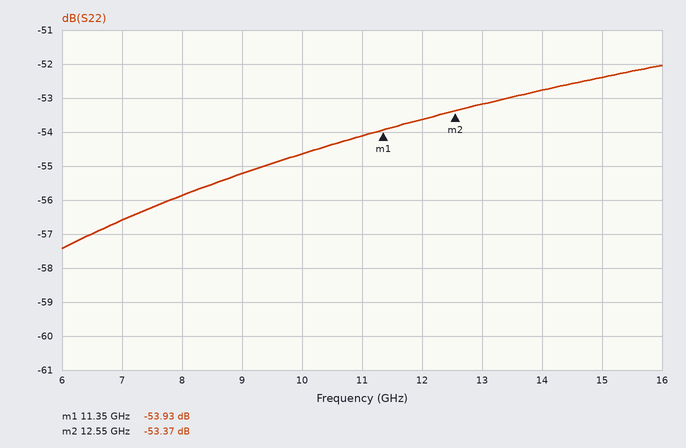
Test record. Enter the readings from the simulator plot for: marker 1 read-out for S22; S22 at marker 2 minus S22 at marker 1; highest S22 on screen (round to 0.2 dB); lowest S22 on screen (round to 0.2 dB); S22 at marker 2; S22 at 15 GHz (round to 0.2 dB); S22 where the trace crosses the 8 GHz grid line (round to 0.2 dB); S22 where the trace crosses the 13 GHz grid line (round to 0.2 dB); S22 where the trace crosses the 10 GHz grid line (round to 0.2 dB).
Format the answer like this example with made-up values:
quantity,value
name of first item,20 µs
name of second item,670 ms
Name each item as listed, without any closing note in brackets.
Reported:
quantity,value
marker 1 read-out for S22,-53.93 dB
S22 at marker 2 minus S22 at marker 1,0.56 dB
highest S22 on screen,-52.0 dB
lowest S22 on screen,-57.4 dB
S22 at marker 2,-53.37 dB
S22 at 15 GHz,-52.4 dB
S22 where the trace crosses the 8 GHz grid line,-55.8 dB
S22 where the trace crosses the 13 GHz grid line,-53.2 dB
S22 where the trace crosses the 10 GHz grid line,-54.6 dB
